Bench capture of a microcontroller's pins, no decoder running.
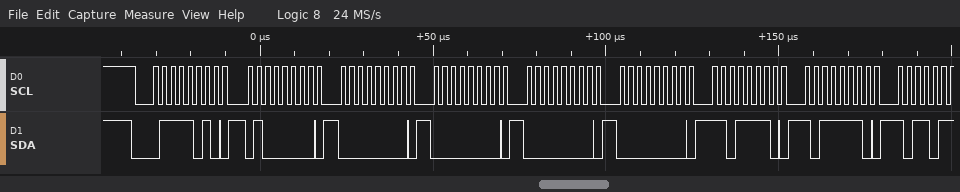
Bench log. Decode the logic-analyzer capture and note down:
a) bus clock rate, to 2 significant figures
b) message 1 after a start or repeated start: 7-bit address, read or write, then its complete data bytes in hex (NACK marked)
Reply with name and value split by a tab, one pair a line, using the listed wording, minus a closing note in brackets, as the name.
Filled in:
bus clock rate, to 2 significant figures	400 kHz
message 1 after a start or repeated start: 7-bit address, read or write, then its complete data bytes in hex	0x3D write: 40 00 00 00 00 DE BE
